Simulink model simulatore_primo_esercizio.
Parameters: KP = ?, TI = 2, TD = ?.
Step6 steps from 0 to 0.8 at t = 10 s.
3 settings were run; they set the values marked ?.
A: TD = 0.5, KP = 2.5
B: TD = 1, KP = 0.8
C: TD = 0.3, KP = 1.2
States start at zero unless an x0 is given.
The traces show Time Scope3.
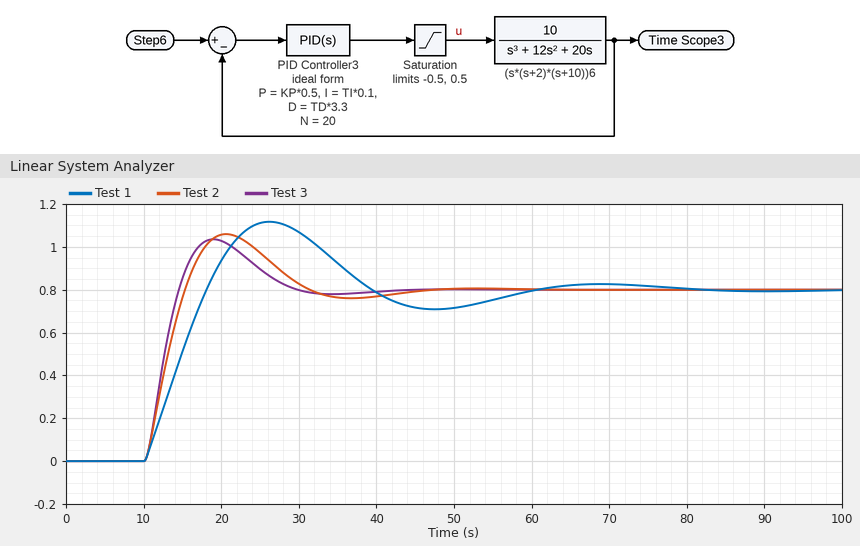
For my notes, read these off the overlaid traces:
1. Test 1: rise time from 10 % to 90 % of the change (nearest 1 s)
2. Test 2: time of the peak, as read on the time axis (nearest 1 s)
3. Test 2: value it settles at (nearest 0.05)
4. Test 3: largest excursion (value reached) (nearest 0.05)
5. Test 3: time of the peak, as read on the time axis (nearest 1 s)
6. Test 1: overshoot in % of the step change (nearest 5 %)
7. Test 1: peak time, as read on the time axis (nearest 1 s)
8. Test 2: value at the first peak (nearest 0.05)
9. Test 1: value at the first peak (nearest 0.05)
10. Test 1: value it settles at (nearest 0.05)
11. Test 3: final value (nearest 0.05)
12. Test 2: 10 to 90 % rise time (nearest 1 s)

6 s
21 s
0.80
1.05
19 s
40 %
26 s
1.05
1.10
0.80
0.80
4 s
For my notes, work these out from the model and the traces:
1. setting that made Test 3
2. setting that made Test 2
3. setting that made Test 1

A
C
B
